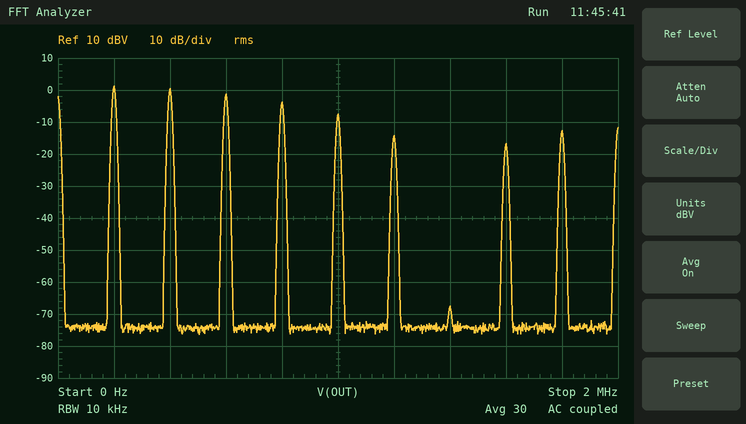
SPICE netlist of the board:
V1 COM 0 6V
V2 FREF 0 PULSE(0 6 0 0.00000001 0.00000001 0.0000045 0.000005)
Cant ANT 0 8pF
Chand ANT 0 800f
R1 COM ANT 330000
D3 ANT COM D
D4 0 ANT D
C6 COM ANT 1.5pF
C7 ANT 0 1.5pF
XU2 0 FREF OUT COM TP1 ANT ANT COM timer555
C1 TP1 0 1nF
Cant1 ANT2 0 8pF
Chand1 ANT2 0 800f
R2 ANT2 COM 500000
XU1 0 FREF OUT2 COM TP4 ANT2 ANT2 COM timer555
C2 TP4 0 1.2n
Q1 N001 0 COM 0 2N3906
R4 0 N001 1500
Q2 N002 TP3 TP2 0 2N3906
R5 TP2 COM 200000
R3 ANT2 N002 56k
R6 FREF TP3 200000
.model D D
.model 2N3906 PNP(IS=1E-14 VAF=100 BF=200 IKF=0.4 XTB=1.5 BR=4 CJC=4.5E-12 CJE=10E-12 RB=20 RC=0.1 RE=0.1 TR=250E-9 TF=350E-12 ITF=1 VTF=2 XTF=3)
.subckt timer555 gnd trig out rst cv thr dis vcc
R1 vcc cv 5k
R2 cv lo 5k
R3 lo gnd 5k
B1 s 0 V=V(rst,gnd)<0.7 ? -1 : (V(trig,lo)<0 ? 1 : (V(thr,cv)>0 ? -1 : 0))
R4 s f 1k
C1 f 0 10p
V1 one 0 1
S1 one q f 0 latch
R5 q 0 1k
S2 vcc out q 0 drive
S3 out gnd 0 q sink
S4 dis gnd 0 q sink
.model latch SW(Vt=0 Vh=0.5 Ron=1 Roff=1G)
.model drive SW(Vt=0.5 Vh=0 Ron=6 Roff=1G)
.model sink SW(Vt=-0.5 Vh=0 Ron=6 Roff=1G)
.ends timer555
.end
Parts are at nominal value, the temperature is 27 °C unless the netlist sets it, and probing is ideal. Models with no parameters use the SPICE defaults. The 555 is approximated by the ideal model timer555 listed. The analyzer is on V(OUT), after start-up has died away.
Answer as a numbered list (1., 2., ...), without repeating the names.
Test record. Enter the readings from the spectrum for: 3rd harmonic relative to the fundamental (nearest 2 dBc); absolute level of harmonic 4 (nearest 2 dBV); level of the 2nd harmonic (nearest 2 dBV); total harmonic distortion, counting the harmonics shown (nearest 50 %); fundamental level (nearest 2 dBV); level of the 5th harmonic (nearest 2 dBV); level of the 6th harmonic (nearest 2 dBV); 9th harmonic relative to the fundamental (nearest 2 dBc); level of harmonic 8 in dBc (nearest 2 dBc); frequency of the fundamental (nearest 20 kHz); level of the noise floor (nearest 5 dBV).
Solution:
1. -2 dBc
2. -4 dBV
3. 0 dBV
4. 150 %
5. 2 dBV
6. -8 dBV
7. -14 dBV
8. -14 dBc
9. -18 dBc
10. 200 kHz
11. -75 dBV
